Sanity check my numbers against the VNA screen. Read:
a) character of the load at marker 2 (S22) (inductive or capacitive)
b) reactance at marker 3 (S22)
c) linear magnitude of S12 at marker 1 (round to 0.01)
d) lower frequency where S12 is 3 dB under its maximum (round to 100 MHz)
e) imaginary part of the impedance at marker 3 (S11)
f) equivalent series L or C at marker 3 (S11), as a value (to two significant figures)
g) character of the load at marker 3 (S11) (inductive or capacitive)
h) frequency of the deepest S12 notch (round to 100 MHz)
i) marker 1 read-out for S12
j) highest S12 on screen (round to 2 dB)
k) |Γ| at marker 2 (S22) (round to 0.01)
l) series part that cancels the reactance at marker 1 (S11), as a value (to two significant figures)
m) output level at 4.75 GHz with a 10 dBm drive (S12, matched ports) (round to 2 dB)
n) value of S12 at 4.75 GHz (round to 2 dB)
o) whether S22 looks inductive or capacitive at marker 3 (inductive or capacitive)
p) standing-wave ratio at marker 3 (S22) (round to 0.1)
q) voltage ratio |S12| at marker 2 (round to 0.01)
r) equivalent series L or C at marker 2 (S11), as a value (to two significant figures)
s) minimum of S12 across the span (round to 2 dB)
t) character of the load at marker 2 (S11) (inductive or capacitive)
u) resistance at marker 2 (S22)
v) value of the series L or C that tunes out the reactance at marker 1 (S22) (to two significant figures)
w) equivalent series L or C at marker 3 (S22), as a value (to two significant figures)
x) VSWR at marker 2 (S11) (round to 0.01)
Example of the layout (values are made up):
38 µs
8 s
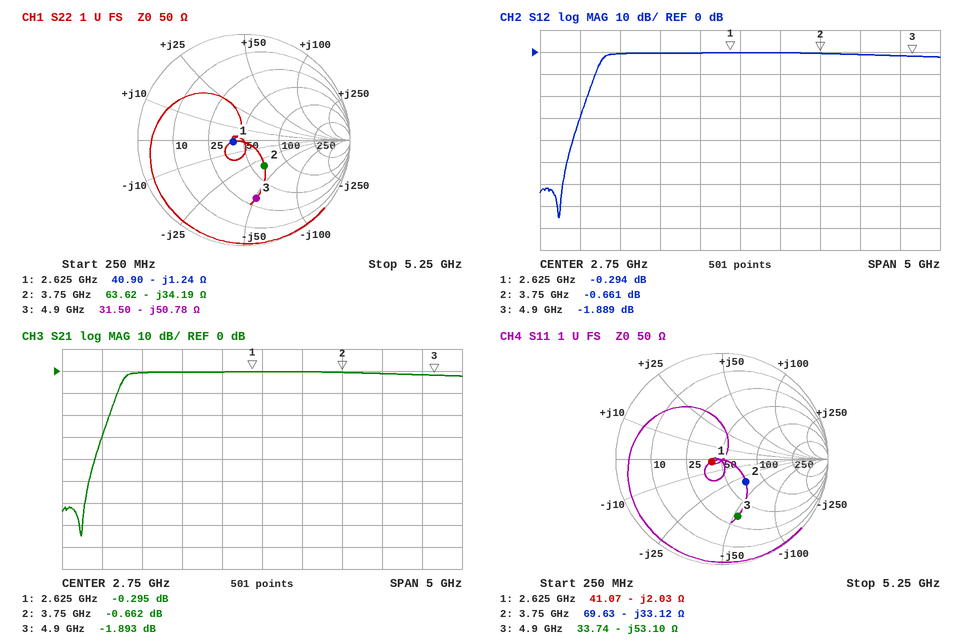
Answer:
capacitive
-50.78 Ω
0.97
1.0 GHz
-53.10 Ω
610 fF
capacitive
500 MHz
-0.294 dB
0 dB
0.31
120 pH
8 dBm
-2 dB
capacitive
3.6
0.93
1.3 pF
-76 dB
capacitive
63.62 Ω
75 pH
640 fF
1.90
